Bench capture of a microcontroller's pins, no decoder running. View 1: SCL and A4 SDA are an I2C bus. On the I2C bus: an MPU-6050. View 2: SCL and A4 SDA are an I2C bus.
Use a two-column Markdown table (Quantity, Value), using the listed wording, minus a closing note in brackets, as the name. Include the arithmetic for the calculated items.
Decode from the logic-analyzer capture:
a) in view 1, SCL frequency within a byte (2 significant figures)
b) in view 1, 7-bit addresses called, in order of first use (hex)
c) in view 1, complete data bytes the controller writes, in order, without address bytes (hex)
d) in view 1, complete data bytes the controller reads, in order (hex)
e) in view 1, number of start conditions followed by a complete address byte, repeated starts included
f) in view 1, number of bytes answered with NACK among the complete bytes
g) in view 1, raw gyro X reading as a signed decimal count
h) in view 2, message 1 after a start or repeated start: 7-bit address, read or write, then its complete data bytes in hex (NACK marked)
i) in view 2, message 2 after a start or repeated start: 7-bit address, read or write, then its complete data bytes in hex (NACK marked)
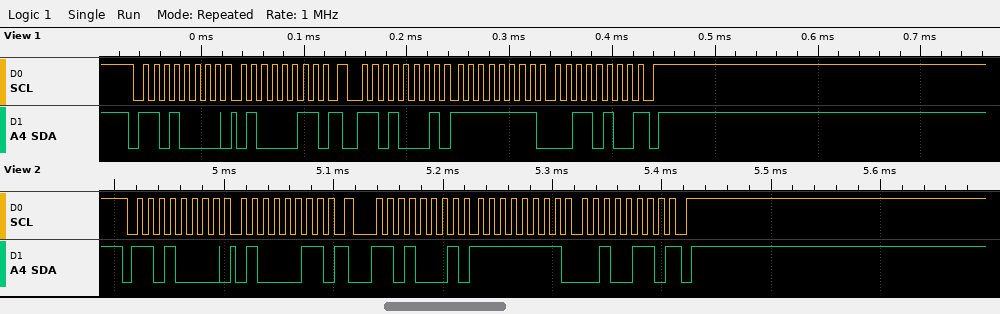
| Quantity | Value |
|---|---|
| in view 1, SCL frequency within a byte | 100 kHz |
| in view 1, 7-bit addresses called, in order of first use | 0x68 |
| in view 1, complete data bytes the controller writes, in order, without address bytes | 43 |
| in view 1, complete data bytes the controller reads, in order | FF 34 |
| in view 1, number of start conditions followed by a complete address byte, repeated starts included | 2 |
| in view 1, number of bytes answered with NACK among the complete bytes | 1 |
| in view 1, raw gyro X reading as a signed decimal count | 0xFF34 = -204 |
| in view 2, message 1 after a start or repeated start: 7-bit address, read or write, then its complete data bytes in hex | 0x68 write: 43 |
| in view 2, message 2 after a start or repeated start: 7-bit address, read or write, then its complete data bytes in hex | 0x68 read: FF 26 NACK |
